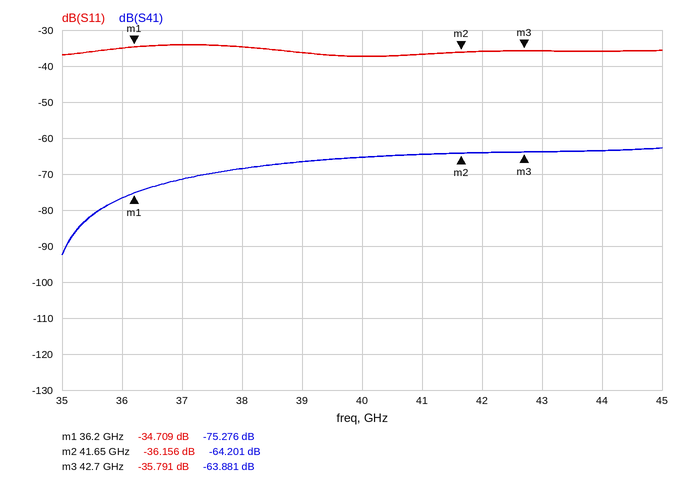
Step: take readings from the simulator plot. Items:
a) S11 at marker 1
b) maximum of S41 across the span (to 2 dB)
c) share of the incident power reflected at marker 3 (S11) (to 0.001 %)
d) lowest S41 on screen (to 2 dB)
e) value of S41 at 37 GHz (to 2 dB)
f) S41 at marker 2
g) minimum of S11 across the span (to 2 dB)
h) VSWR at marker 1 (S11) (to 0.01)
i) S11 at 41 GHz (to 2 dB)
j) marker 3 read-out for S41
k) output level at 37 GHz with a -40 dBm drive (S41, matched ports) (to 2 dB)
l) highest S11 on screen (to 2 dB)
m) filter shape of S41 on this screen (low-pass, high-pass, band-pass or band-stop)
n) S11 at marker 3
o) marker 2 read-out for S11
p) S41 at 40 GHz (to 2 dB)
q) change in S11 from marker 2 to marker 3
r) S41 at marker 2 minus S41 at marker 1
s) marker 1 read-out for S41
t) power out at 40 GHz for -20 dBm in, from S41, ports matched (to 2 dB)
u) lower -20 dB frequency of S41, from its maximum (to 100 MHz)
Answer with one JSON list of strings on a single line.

["-34.709 dB", "-62 dB", "0.026 %", "-92 dB", "-72 dB", "-64.201 dB", "-38 dB", "1.04", "-36 dB", "-63.881 dB", "-112 dBm", "-34 dB", "high-pass", "-35.791 dB", "-36.156 dB", "-66 dB", "0.365 dB", "11.075 dB", "-75.276 dB", "-86 dBm", "35.4 GHz"]
